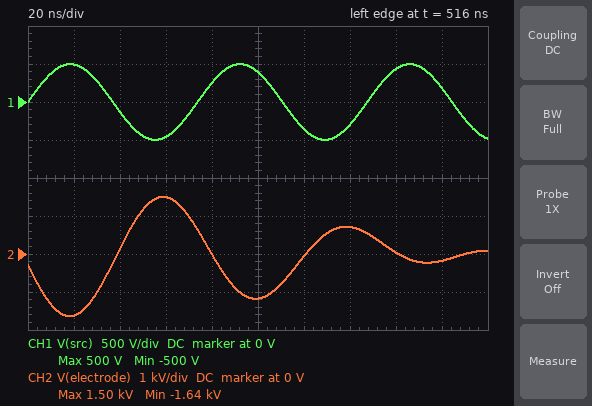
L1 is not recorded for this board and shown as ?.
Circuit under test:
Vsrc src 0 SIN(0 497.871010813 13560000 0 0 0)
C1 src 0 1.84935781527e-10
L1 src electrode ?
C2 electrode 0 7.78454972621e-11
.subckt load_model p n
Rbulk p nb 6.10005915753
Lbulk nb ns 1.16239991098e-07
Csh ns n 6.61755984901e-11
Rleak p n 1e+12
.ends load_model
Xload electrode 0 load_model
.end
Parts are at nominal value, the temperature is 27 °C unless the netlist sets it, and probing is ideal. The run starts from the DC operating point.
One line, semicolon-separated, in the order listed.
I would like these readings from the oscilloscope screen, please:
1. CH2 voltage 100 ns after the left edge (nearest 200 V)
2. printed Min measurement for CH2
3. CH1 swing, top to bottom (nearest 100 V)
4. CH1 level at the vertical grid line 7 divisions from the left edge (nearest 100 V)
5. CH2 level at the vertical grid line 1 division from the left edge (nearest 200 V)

-1.2 kV; -1.64 kV; 1.0 kV; -300 V; -1.6 kV
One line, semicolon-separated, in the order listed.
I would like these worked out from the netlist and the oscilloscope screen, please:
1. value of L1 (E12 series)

1.5 µH
